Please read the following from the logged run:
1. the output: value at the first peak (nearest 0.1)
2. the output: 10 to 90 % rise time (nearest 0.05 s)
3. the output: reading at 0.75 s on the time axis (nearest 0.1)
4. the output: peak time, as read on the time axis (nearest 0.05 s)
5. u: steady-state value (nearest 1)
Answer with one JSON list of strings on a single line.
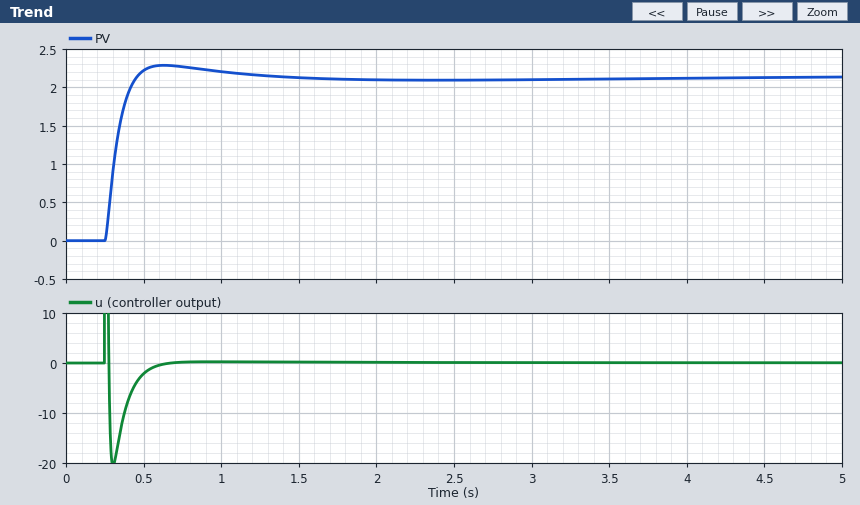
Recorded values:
["2.3", "0.15 s", "2.3", "0.65 s", "0"]
